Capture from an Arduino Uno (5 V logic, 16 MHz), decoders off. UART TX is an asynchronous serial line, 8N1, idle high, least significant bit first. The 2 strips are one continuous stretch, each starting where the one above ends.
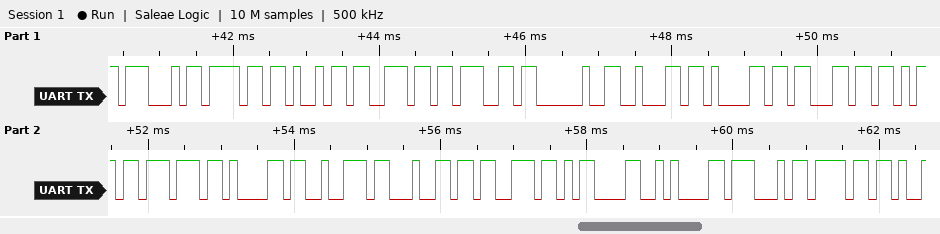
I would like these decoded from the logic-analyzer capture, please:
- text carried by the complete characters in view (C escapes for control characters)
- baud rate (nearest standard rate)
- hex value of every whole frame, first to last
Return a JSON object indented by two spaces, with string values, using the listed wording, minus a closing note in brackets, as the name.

{
  "text carried by the complete characters in view": "\"Going backwards\\r\\nGo\"",
  "baud rate": "9600 baud",
  "hex value of every whole frame, first to last": "0x47 0x6F 0x69 0x6E 0x67 0x20 0x62 0x61 0x63 0x6B 0x77 0x61 0x72 0x64 0x73 0x0D 0x0A 0x47 0x6F"
}
